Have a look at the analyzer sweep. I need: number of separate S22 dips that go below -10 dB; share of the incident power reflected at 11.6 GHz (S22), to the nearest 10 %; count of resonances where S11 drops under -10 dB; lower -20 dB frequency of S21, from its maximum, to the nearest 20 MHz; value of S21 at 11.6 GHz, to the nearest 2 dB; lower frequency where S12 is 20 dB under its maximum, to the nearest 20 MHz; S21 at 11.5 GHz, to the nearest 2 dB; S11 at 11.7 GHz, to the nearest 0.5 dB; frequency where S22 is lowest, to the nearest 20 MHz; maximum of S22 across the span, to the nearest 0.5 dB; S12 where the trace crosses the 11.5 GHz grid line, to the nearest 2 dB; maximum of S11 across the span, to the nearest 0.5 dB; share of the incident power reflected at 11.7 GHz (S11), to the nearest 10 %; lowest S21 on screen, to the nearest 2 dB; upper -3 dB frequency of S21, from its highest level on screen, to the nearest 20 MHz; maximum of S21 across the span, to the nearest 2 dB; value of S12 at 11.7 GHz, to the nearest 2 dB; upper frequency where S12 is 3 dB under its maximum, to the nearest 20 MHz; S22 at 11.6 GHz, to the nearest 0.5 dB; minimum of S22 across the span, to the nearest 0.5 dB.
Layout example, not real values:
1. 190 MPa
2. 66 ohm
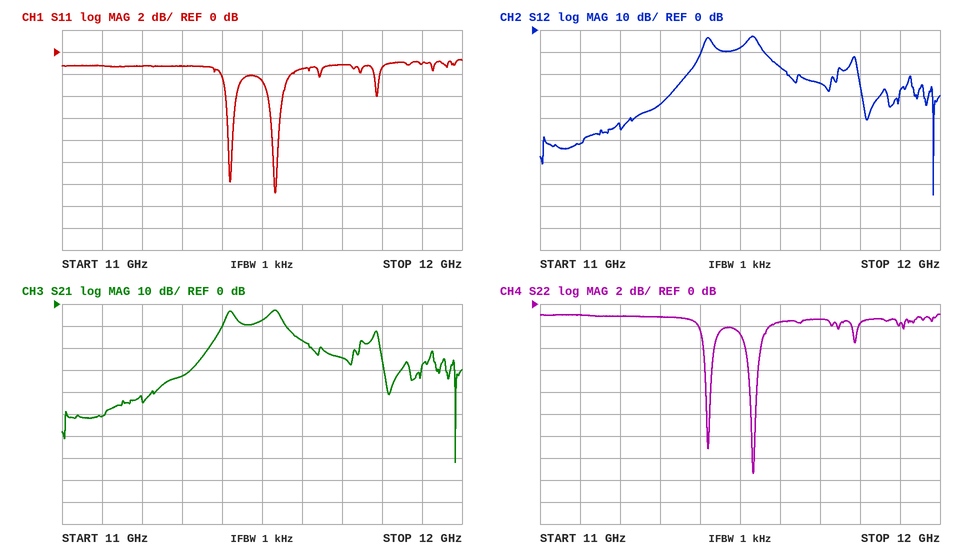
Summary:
1. 2
2. 70 %
3. 2
4. 11.36 GHz
5. -16 dB
6. 11.36 GHz
7. -8 dB
8. -1.0 dB
9. 11.54 GHz
10. -1.0 dB
11. -8 dB
12. -0.5 dB
13. 80 %
14. -72 dB
15. 11.54 GHz
16. -2 dB
17. -24 dB
18. 11.54 GHz
19. -1.5 dB
20. -15.5 dB
